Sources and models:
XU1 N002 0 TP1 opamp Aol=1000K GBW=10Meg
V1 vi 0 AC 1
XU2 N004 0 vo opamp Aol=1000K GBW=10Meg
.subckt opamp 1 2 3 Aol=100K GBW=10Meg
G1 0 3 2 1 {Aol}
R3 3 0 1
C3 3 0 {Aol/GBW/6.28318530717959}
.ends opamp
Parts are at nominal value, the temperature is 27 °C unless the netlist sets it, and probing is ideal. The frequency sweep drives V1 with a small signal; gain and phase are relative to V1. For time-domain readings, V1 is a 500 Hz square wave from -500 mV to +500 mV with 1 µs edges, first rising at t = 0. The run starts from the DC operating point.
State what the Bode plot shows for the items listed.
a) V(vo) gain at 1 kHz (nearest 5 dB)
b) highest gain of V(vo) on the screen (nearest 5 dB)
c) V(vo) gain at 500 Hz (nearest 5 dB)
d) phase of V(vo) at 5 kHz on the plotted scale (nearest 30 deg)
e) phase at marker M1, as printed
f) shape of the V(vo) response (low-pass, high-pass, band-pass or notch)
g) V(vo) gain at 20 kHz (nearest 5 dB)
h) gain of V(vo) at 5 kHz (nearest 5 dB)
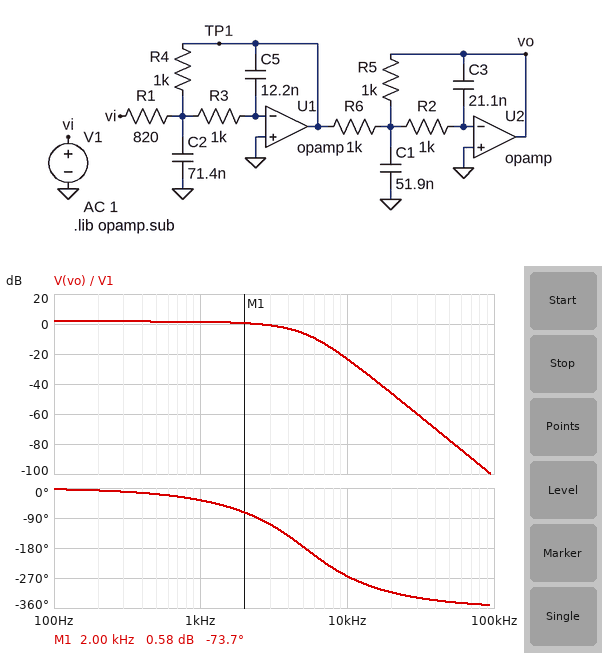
0 dB
0 dB
0 dB
-180 deg
-73.7 deg
low-pass
-45 dB
-5 dB
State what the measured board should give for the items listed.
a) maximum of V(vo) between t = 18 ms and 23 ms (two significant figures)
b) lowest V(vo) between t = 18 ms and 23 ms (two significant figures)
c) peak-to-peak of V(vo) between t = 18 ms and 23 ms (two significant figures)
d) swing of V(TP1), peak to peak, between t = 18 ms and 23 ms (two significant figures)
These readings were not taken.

620 mV
-620 mV
1.2 V
1.4 V
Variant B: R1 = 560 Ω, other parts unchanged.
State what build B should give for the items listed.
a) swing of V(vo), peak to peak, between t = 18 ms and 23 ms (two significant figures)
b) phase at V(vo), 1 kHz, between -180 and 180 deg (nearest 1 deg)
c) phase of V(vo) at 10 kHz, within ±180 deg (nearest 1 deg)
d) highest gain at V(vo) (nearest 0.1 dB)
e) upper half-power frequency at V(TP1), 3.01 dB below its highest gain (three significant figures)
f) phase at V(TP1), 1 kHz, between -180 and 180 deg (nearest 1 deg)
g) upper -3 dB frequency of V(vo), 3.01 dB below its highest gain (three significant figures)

1.8 V
-39 deg
100 deg
5.0 dB
4.82 kHz
163 deg
2.80 kHz
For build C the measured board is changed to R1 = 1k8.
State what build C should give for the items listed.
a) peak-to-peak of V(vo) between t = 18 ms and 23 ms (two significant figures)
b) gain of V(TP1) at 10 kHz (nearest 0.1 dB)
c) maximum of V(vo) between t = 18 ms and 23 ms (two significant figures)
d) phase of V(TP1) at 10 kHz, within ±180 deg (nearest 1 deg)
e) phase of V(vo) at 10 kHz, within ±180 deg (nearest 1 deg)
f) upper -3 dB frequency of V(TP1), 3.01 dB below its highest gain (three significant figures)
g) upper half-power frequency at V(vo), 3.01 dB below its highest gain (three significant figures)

580 mV
-15.0 dB
290 mV
39 deg
89 deg
6.24 kHz
3.85 kHz
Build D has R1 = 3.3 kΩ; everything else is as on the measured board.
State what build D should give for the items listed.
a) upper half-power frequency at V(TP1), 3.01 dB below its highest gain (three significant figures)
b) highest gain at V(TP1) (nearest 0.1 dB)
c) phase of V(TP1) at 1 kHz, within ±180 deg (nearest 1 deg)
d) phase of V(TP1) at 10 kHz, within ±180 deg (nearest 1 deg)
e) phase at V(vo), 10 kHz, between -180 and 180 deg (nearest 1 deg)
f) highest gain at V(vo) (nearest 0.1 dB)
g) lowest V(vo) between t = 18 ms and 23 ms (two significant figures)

6.34 kHz
-8.8 dB
170 deg
36 deg
86 deg
-10.4 dB
-160 mV
